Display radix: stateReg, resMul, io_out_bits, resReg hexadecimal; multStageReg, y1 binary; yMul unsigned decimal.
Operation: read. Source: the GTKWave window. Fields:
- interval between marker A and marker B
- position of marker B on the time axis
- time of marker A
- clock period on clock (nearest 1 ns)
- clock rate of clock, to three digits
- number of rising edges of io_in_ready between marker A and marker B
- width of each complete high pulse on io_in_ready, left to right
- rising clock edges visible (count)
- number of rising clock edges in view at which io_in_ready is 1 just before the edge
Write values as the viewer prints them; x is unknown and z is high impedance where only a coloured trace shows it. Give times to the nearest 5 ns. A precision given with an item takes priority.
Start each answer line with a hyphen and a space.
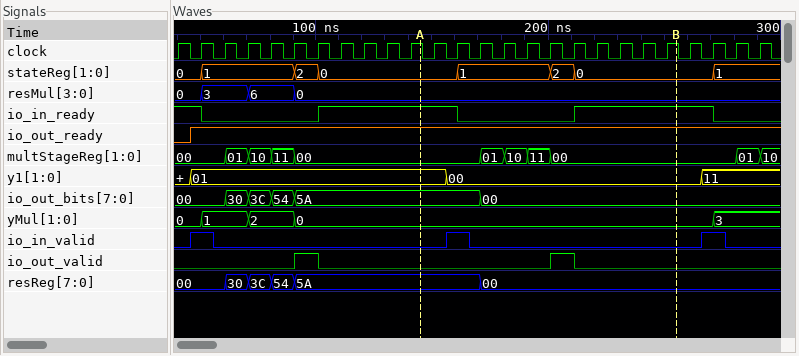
- 110 ns
- 255 ns
- 145 ns
- 10 ns
- 100 MHz
- 1
- 60 ns, 60 ns
- 26
- 14
